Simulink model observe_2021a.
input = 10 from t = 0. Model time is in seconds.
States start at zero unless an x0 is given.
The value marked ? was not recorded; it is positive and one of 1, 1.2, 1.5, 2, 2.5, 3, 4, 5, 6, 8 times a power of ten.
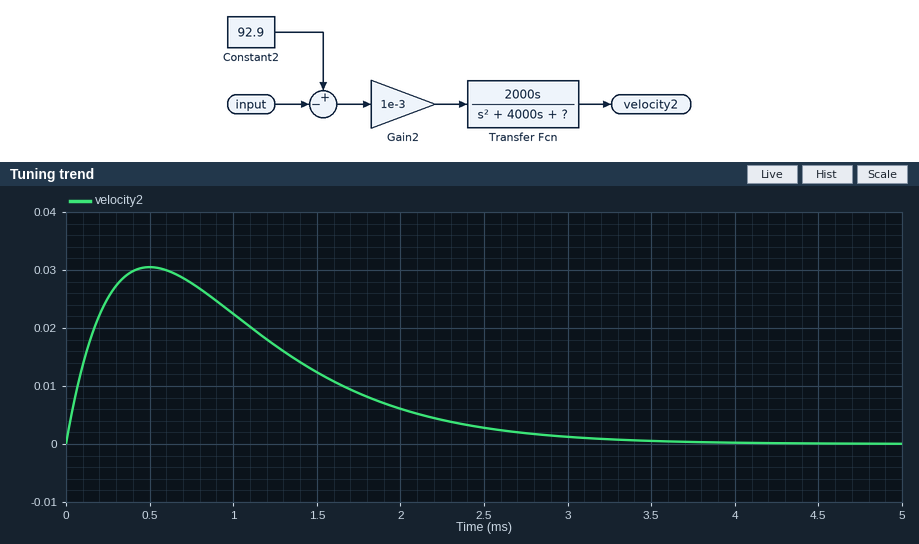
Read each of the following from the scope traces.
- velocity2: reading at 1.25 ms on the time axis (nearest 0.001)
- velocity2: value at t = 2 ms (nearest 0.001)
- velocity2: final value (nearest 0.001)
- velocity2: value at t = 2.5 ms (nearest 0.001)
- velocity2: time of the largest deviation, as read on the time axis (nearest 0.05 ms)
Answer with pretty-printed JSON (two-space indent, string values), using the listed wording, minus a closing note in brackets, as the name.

{
  "velocity2: reading at 1.25 ms on the time axis": "0.017",
  "velocity2: value at t = 2 ms": "0.006",
  "velocity2: final value": "0.000",
  "velocity2: value at t = 2.5 ms": "0.003",
  "velocity2: time of the largest deviation, as read on the time axis": "0.50 ms"
}
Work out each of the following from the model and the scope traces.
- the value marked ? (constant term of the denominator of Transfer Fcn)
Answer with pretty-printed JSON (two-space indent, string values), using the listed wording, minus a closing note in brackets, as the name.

{
  "the value marked ?": "4e+06"
}
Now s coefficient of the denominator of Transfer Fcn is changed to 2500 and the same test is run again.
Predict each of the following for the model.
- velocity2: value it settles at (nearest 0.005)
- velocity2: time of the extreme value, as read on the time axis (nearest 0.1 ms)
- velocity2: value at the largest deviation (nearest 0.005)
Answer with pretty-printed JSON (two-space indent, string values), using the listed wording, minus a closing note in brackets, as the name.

{
  "velocity2: value it settles at": "0.000",
  "velocity2: time of the extreme value, as read on the time axis": "0.6 ms",
  "velocity2: value at the largest deviation": "0.040"
}
